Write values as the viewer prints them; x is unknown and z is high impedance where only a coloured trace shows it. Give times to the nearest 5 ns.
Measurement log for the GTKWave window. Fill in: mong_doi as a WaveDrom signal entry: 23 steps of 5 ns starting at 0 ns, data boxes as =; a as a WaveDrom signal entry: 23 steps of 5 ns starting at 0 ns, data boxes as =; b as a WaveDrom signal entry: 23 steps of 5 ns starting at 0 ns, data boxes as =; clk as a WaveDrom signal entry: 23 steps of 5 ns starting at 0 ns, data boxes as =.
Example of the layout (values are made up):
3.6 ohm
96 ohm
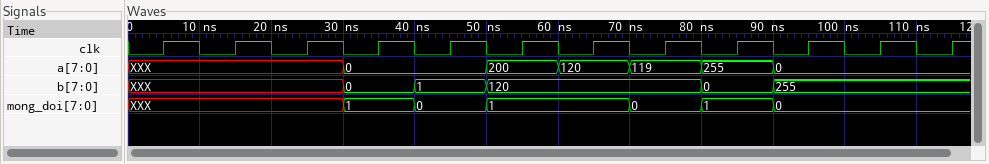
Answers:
{name: 'mong_doi', wave: 'x.....=.=.=...=.=.=....', data: '1 0 1 0 1 0'}
{name: 'a', wave: 'x.....=...=.=.=.=.=....', data: '0 200 120 119 255 0'}
{name: 'b', wave: 'x.....=.=.=.....=.=....', data: '0 1 120 0 255'}
{name: 'clk', wave: '01010101010101010101010'}
